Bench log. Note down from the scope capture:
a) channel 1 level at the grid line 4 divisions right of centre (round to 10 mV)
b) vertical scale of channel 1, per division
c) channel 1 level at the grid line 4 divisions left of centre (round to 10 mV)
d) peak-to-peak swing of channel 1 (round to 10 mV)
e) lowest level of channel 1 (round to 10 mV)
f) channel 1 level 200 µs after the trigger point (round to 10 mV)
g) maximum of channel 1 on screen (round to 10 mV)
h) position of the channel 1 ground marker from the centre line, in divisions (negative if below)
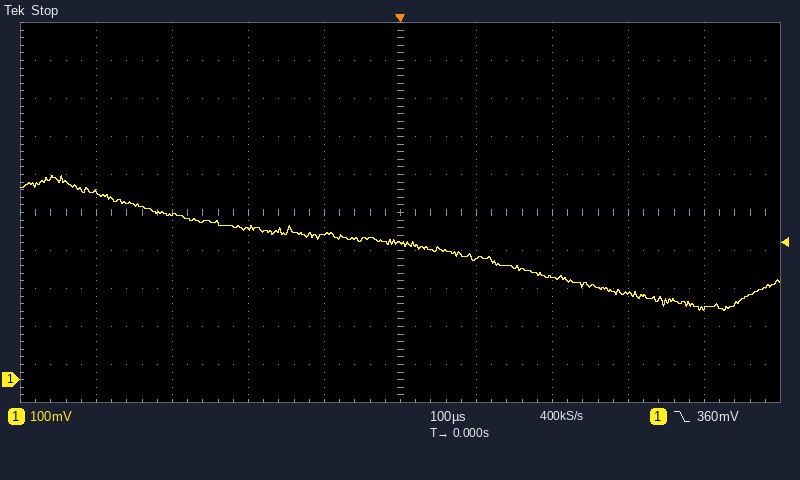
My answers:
190 mV
100 mV
490 mV
360 mV
180 mV
270 mV
540 mV
-4.4 div
